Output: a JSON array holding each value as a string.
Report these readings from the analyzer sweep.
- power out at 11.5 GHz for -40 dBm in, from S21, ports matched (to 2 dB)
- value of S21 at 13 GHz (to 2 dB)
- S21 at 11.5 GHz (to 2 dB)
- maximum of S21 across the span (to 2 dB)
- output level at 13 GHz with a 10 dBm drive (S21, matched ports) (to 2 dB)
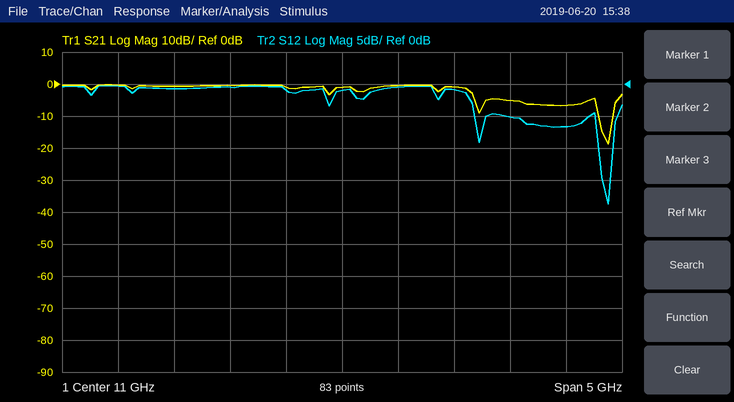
["-40 dBm", "-6 dB", "0 dB", "0 dB", "4 dBm"]
